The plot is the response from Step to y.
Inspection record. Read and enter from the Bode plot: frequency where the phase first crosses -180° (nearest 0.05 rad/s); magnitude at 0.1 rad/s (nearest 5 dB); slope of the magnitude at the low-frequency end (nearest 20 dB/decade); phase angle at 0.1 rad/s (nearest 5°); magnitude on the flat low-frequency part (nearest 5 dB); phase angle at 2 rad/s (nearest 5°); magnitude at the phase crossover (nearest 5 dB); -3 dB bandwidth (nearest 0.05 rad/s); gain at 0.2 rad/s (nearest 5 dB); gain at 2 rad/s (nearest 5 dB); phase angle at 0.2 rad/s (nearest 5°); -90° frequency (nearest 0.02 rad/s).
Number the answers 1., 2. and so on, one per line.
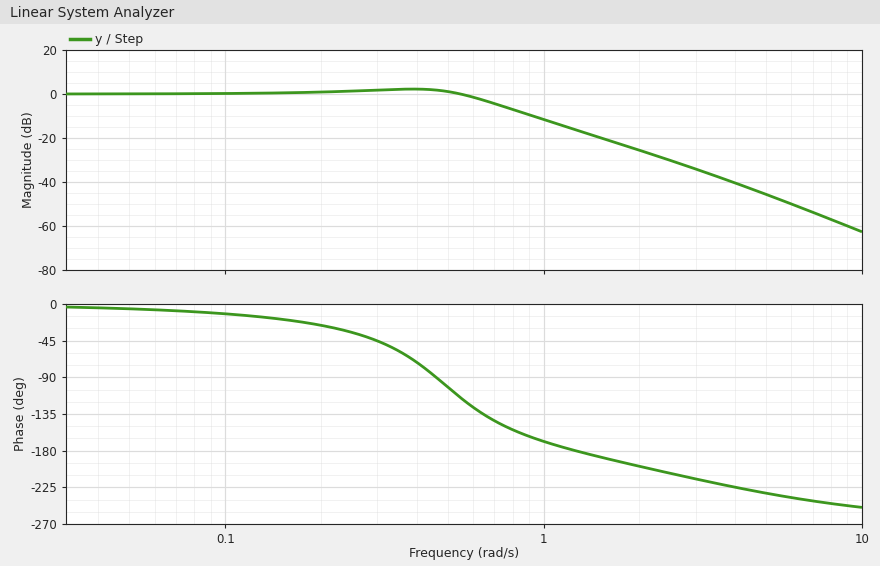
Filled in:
1. 1.25 rad/s
2. 0 dB
3. 0 dB/decade
4. -10°
5. 0 dB
6. -200°
7. -15 dB
8. 0.65 rad/s
9. 0 dB
10. -25 dB
11. -25°
12. 0.46 rad/s
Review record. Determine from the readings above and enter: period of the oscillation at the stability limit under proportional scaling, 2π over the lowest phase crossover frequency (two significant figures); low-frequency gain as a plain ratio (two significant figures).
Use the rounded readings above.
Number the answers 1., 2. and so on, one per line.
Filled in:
1. 5.0 s
2. 1.0
